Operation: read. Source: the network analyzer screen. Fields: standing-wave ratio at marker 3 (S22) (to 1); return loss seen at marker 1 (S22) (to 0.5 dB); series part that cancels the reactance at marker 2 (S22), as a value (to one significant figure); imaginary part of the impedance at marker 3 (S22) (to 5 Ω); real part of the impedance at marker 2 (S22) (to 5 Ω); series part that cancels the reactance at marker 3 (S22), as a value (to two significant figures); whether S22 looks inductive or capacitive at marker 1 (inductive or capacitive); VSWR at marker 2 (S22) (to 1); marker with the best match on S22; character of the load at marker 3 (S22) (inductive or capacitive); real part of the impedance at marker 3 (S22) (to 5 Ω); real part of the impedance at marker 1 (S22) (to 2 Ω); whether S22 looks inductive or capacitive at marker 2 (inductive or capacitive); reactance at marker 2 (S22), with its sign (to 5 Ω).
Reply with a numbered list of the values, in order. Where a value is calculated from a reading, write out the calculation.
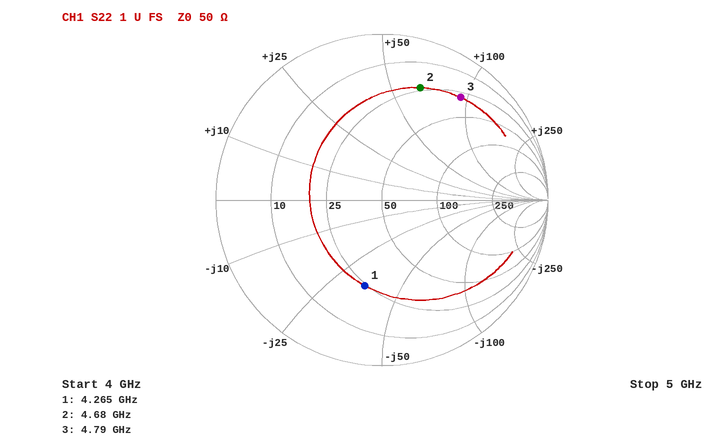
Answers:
1. 8
2. 5.5 dB
3. C = 1/(2π × 4.68 GHz × 65 Ω) ≈ 523 fF, so 500 fF to one significant figure
4. +95 Ω
5. 25 Ω
6. C = 1/(2π × 4.79 GHz × 95 Ω) ≈ 350 fF
7. capacitive
8. 6
9. marker 1
10. inductive
11. 30 Ω
12. 24 Ω
13. inductive
14. +65 Ω
